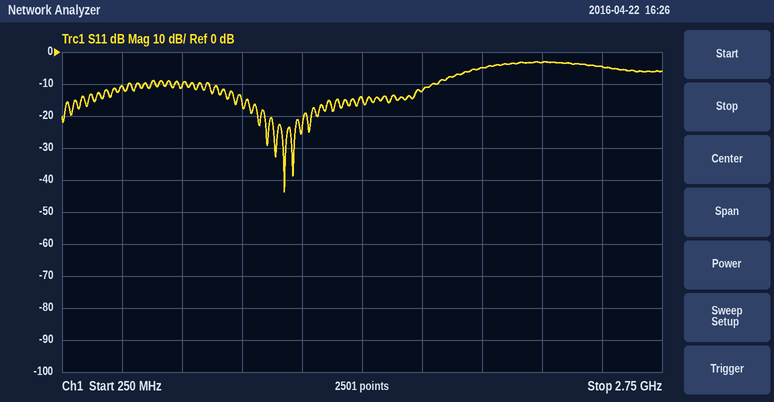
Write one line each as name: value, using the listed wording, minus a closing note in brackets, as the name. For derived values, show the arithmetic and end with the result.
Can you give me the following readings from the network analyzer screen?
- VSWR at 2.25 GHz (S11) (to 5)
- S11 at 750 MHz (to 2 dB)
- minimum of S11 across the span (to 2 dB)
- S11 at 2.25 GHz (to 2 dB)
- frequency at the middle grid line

VSWR at 2.25 GHz (S11): |Γ| = 10^(-4/20) = 0.6310; VSWR = (1 + 0.6310)/(1 − 0.6310) ≈ 4.42, so 5 to the nearest 5
S11 at 750 MHz: -10 dB
minimum of S11 across the span: -44 dB
S11 at 2.25 GHz: -4 dB
frequency at the middle grid line: 1.5 GHz
